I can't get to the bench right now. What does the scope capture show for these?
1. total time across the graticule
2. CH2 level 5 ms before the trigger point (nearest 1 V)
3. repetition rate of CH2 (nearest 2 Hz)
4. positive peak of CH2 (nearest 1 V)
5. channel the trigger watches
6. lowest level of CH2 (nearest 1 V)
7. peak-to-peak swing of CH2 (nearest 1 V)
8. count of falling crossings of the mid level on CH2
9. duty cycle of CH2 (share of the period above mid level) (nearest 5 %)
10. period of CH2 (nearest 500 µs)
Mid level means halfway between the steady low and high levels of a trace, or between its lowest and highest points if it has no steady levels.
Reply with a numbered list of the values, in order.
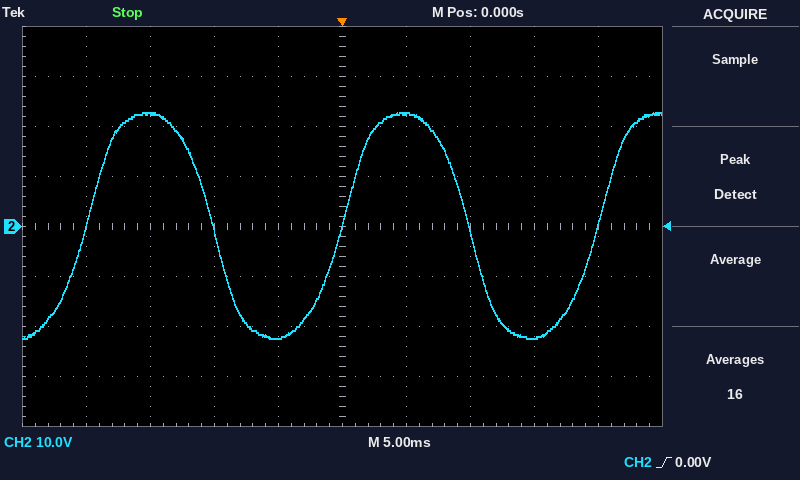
1. 50 ms
2. -22 V
3. 50 Hz
4. 23 V
5. CH2
6. -22 V
7. 45 V
8. 2
9. 50 %
10. 20.0 ms
